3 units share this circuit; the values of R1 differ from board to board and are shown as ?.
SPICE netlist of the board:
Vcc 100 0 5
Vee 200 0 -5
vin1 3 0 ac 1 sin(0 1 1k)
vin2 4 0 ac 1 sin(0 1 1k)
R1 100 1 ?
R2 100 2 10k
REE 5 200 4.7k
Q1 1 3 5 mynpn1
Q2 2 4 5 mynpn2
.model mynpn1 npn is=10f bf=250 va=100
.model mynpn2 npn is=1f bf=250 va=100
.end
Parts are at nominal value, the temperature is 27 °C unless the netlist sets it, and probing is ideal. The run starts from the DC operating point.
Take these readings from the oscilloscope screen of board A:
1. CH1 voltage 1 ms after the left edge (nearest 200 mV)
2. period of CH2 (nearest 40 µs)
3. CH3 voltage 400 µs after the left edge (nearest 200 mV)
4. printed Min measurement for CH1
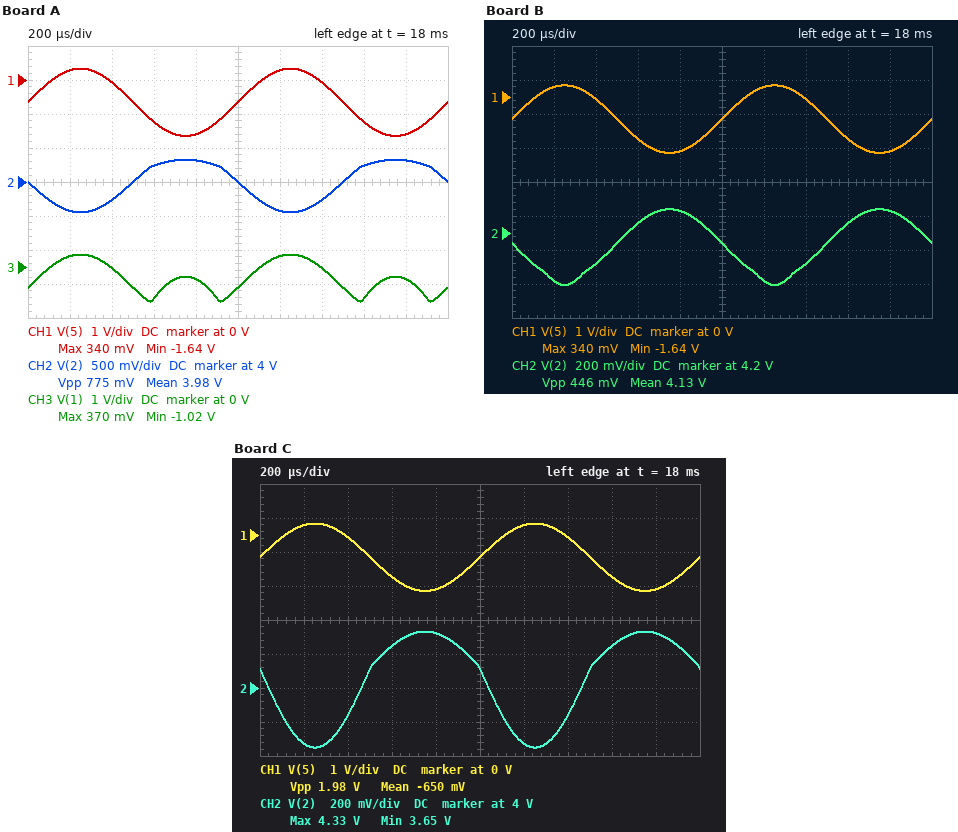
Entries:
-600 mV
1.00 ms
0 V
-1.64 V
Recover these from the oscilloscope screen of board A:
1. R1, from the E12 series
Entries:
8.2 kΩ
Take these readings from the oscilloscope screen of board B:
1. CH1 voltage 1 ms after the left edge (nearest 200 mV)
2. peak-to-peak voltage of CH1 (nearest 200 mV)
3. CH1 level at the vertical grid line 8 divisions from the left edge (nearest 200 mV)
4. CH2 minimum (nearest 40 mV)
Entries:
-600 mV
2.0 V
-1.2 V
3.88 V
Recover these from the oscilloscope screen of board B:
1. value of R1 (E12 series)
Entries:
4.7 kΩ
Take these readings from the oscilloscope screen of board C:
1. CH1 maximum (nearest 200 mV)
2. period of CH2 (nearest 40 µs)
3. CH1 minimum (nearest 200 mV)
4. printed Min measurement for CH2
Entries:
400 mV
1.00 ms
-1.6 V
3.65 V
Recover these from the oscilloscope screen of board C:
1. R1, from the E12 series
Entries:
6.8 kΩ
